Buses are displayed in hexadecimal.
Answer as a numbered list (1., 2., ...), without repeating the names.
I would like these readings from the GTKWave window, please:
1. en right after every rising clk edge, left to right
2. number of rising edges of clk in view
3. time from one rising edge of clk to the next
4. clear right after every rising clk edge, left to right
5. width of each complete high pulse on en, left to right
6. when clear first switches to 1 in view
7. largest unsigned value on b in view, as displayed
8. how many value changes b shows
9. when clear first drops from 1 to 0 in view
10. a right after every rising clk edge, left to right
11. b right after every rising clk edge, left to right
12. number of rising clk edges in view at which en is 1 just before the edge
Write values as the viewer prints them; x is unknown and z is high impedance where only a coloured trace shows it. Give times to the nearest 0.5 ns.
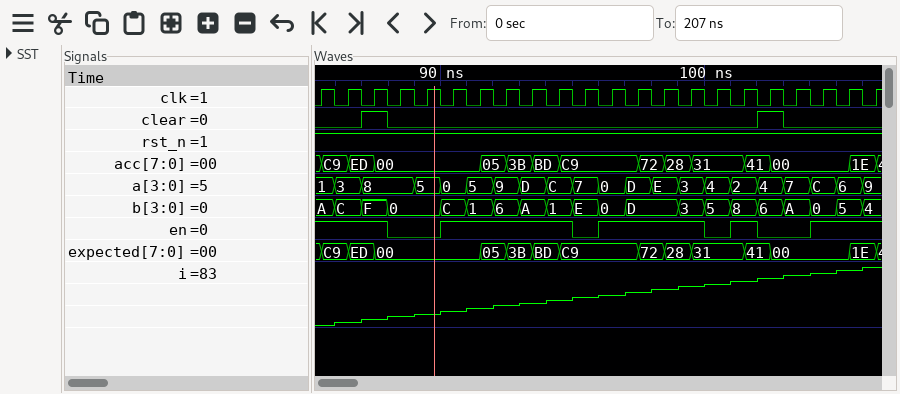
1. 1 1 1 0 0 1 1 1 1 1 0 1 1 1 1 0 1 0 0 1 1 1
2. 22
3. 1 ns
4. 0 0 1 0 0 0 0 0 0 0 0 0 0 0 0 0 0 1 0 0 0 0
5. 5 ns, 4 ns, 1 ns
6. 87 ns
7. F
8. 19
9. 88 ns
10. 1, 3, 8, 8, 5, 0, 5, 9, D, C, 7, 0, D, E, 3, 4, 2, 4, 7, C, 6, 9
11. A, C, F, 0, 0, C, 1, 6, A, 1, E, 0, D, D, 3, 5, 8, 6, A, 0, 5, 4
12. 16
